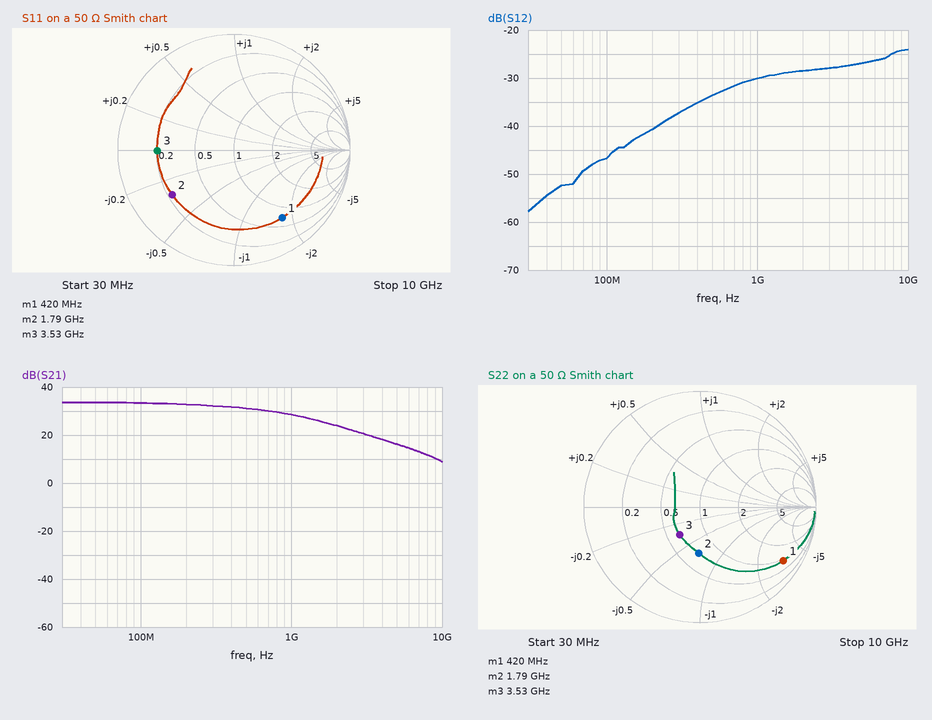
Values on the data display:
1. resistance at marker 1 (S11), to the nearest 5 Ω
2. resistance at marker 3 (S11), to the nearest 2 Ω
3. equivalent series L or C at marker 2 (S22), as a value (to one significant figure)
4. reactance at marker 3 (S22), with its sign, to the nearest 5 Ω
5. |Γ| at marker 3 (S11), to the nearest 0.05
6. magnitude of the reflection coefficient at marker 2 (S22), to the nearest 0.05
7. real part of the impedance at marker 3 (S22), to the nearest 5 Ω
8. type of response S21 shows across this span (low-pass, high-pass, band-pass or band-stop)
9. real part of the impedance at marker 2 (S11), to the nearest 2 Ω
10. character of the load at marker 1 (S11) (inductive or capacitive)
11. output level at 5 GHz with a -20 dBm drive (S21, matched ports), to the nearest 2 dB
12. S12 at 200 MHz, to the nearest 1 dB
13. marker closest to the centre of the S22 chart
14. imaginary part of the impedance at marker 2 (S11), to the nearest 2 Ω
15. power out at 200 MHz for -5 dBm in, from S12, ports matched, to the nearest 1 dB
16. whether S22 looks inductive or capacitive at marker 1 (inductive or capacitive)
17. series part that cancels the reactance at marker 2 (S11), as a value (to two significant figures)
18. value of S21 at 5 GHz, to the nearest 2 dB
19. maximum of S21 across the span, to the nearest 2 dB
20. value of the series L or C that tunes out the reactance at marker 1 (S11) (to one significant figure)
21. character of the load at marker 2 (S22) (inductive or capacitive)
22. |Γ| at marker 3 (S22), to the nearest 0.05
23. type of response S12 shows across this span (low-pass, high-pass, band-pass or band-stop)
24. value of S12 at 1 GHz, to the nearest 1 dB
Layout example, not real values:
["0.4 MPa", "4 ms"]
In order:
["35 Ω", "10 Ω", "3 pF", "-15 Ω", "0.65", "0.40", "30 Ω", "low-pass", "12 Ω", "capacitive", "-4 dBm", "-41 dB", "marker 3", "-16 Ω", "-46 dBm", "capacitive", "1.4 nH", "16 dB", "34 dB", "30 nH", "capacitive", "0.30", "high-pass", "-30 dB"]
